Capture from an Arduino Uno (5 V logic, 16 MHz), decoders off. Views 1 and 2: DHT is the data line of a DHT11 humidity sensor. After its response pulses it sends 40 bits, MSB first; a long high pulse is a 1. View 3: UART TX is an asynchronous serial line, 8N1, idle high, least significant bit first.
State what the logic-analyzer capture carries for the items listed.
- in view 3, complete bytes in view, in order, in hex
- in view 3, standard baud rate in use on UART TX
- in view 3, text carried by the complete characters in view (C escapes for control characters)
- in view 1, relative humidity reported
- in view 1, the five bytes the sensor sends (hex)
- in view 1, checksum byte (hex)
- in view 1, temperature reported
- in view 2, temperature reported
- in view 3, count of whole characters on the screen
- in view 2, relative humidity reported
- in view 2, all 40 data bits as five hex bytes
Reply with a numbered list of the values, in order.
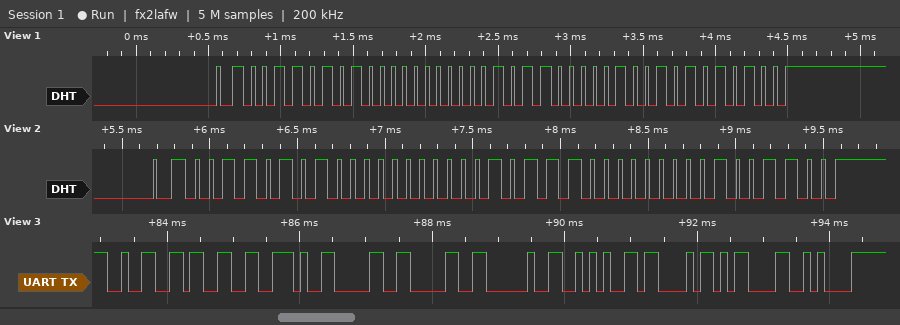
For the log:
1. 32 33 2E 30 30 20 2A 43 0D 0A
2. 9600 baud
3. "23.00 *C\r\n"
4. 53 %
5. 35 00 16 09 54
6. 0x54
7. 22.9 °C
8. 23.0 °C
9. 10
10. 53 %
11. 35 00 17 00 4C
